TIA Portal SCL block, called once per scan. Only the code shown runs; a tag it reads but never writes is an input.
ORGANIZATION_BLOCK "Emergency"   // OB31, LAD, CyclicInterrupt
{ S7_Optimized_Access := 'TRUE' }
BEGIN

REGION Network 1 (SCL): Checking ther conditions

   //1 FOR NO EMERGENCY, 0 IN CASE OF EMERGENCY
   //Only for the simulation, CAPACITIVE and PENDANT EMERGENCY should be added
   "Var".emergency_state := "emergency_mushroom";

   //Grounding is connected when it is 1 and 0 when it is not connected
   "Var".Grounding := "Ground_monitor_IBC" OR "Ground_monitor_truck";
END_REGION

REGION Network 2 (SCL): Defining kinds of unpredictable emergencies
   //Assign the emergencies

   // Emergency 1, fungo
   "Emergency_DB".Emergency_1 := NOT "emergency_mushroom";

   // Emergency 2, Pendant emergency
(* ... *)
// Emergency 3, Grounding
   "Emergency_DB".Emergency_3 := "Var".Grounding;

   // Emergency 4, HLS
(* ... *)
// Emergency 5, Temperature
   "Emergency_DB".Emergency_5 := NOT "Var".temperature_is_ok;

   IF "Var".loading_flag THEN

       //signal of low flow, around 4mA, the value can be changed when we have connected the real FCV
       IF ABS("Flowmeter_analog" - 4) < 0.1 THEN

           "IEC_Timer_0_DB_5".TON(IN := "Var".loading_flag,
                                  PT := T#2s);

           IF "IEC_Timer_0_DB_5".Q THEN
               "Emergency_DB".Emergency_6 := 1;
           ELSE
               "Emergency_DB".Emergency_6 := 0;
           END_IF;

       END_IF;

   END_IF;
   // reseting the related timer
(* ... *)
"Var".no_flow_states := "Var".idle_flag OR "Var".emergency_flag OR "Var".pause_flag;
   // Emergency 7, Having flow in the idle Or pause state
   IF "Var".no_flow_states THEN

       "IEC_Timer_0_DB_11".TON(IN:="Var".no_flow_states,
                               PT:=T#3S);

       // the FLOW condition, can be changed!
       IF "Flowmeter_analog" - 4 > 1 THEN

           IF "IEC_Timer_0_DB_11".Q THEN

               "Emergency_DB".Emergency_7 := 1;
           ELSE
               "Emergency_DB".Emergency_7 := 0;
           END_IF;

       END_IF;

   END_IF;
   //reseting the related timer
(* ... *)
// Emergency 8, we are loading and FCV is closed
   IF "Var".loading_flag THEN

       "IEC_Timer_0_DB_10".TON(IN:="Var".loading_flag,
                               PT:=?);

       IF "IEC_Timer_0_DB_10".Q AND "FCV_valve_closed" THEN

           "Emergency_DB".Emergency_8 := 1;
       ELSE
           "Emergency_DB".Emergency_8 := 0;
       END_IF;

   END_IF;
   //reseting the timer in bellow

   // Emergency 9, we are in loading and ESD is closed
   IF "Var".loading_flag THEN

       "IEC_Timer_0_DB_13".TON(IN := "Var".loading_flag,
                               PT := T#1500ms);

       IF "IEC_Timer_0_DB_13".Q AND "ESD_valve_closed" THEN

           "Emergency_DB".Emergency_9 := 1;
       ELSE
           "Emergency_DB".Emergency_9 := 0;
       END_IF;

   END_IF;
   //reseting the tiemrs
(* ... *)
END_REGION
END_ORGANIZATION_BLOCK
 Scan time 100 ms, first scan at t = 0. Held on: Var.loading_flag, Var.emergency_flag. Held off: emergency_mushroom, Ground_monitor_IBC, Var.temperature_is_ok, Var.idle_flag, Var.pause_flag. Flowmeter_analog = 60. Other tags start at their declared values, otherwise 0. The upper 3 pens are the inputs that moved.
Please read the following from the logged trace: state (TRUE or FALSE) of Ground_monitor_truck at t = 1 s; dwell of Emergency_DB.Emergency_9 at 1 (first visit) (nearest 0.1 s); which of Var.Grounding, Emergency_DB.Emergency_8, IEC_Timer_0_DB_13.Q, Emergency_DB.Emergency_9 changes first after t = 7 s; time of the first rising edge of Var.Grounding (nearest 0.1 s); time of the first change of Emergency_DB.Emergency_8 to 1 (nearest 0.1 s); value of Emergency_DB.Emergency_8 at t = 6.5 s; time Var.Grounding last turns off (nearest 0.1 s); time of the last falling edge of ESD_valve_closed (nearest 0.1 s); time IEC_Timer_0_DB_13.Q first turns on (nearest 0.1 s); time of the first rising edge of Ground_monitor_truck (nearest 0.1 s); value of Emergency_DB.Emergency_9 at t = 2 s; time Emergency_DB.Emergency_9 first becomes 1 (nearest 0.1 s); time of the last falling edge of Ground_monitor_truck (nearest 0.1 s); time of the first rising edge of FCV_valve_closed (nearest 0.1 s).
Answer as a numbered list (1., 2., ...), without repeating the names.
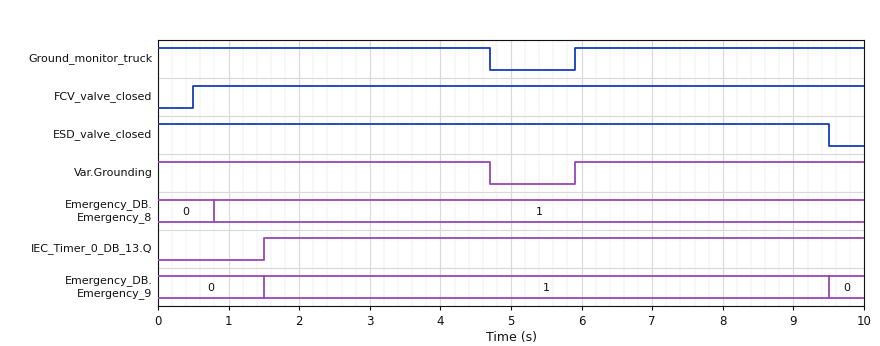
1. TRUE
2. 8.0 s
3. Emergency_DB.Emergency_9
4. 5.9 s
5. 0.8 s
6. 1
7. 4.7 s
8. 9.5 s
9. 1.5 s
10. 5.9 s
11. 1
12. 1.5 s
13. 4.7 s
14. 0.5 s
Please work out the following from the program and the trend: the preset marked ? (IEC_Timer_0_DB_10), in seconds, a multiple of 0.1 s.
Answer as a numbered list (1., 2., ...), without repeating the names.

1. 0.8 s
